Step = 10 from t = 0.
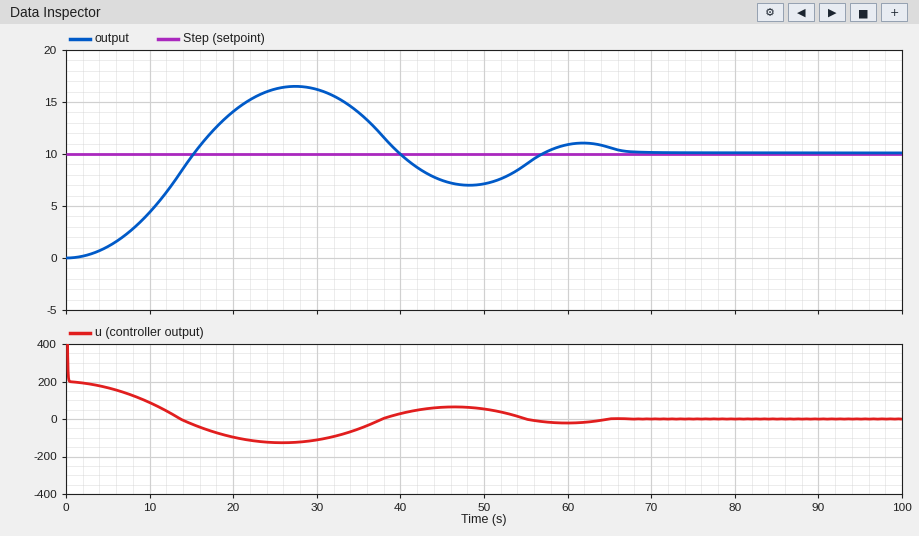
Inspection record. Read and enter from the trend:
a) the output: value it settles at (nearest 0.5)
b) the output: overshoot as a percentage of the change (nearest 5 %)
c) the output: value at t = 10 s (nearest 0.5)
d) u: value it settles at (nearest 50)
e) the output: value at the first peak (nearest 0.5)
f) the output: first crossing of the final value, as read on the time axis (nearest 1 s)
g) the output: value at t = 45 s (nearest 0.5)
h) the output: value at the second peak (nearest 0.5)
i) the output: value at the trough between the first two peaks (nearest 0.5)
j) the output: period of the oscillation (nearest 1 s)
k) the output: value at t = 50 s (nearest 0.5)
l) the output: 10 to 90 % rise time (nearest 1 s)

10.0
65 %
4.5
0
16.5
15 s
7.5
11.0
7.0
34 s
7.0
10 s
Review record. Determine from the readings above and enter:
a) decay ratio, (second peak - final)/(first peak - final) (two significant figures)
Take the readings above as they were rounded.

0.15
